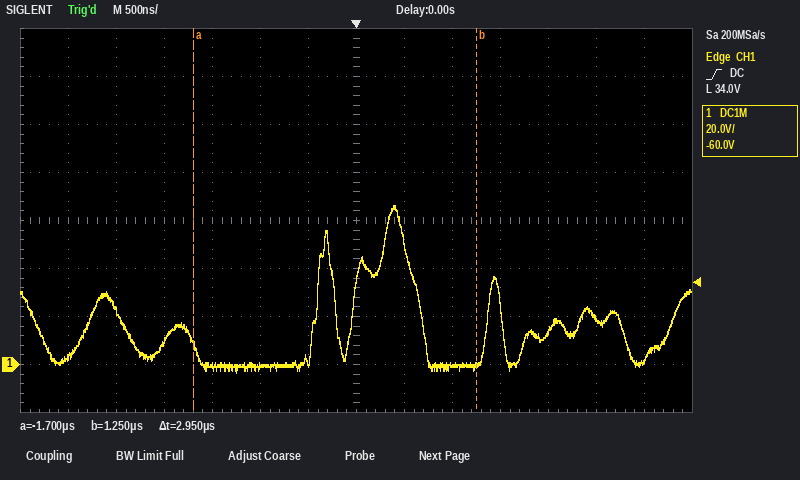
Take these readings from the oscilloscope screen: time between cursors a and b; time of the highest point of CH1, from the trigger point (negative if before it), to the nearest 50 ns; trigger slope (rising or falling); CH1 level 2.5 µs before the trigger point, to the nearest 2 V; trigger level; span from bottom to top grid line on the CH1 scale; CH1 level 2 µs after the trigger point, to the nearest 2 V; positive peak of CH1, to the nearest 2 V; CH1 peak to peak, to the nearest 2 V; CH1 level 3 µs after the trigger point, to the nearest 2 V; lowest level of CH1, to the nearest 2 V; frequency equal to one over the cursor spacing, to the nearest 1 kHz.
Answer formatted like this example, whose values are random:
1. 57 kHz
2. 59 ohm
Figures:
1. 2.95 µs
2. +400 ns
3. rising
4. 22 V
5. 34.0 V
6. 160 V
7. 14 V
8. 66 V
9. 70 V
10. 2 V
11. -4 V
12. 339 kHz
